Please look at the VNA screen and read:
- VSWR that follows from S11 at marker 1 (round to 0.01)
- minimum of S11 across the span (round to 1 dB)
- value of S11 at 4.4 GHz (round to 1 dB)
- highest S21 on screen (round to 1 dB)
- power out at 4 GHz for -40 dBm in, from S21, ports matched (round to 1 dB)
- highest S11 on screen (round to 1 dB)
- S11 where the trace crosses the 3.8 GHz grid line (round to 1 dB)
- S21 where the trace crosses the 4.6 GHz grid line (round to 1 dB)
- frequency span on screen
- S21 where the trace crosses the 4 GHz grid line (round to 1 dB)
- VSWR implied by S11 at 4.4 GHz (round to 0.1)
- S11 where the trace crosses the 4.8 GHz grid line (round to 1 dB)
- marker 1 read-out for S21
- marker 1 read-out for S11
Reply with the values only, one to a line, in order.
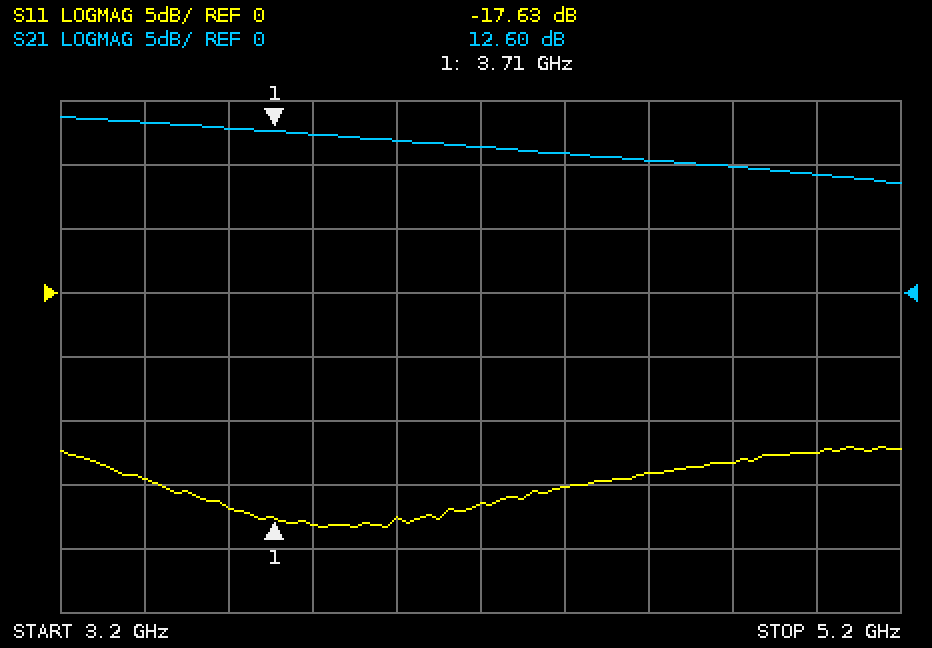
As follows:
1.30
-18 dB
-15 dB
14 dB
-28 dBm
-12 dB
-18 dB
10 dB
2 GHz
12 dB
1.4
-13 dB
12.60 dB
-17.63 dB
